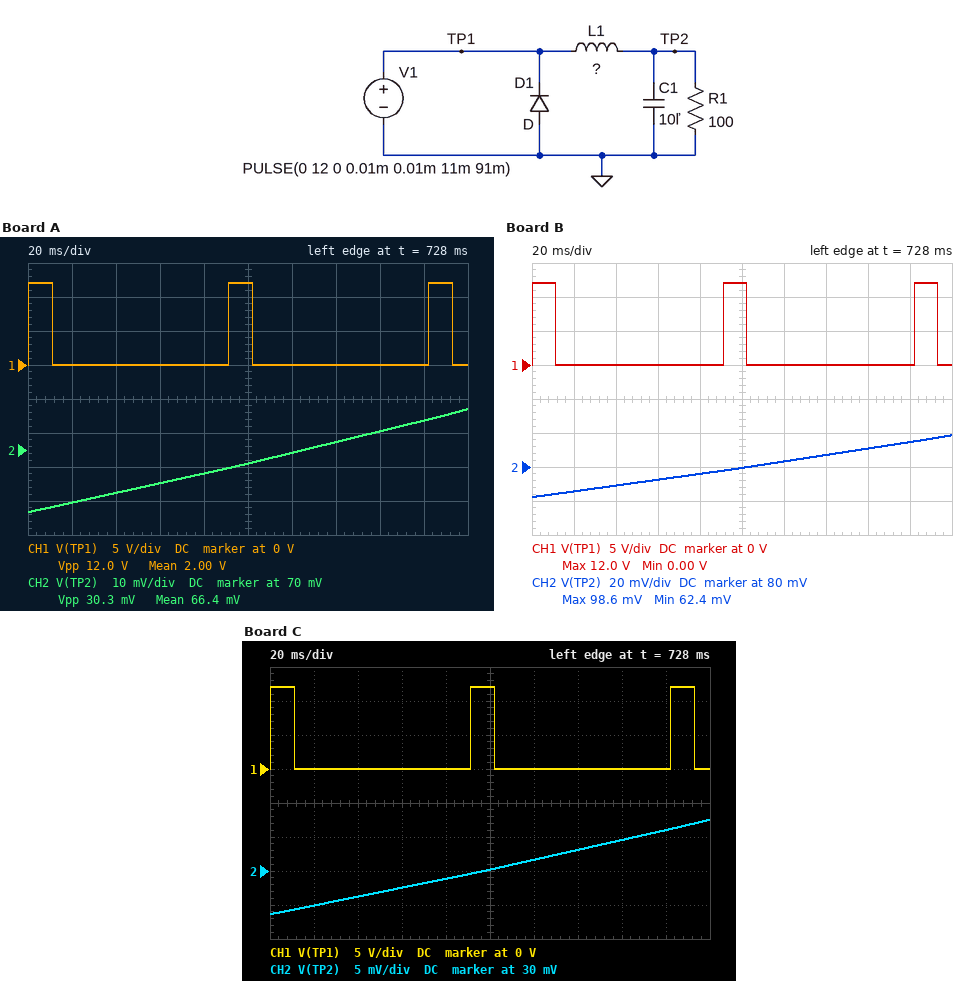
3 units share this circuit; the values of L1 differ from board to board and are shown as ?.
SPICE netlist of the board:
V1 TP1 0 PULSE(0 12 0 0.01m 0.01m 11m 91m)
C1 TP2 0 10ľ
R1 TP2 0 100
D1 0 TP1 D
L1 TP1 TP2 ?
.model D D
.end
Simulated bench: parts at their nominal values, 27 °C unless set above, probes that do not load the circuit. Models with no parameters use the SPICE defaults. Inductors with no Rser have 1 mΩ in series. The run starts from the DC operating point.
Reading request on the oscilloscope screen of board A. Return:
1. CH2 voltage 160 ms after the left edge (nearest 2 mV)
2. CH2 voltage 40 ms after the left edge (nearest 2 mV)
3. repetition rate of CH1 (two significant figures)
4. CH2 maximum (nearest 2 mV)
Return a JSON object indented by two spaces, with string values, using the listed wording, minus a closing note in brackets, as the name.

{
  "CH2 voltage 160 ms after the left edge": "76 mV",
  "CH2 voltage 40 ms after the left edge": "58 mV",
  "repetition rate of CH1": "11 Hz",
  "CH2 maximum": "82 mV"
}
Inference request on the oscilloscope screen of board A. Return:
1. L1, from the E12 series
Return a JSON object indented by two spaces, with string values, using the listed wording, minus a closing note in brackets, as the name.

{
  "L1, from the E12 series": "820 mH"
}
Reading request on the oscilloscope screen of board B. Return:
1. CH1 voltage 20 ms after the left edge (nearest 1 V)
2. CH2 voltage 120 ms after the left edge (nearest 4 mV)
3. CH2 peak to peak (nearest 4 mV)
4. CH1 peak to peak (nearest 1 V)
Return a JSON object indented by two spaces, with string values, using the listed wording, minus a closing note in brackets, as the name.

{
  "CH1 voltage 20 ms after the left edge": "0 V",
  "CH2 voltage 120 ms after the left edge": "84 mV",
  "CH2 peak to peak": "36 mV",
  "CH1 peak to peak": "12 V"
}
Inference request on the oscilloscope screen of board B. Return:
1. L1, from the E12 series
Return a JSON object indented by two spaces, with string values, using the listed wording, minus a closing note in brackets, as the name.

{
  "L1, from the E12 series": "680 mH"
}
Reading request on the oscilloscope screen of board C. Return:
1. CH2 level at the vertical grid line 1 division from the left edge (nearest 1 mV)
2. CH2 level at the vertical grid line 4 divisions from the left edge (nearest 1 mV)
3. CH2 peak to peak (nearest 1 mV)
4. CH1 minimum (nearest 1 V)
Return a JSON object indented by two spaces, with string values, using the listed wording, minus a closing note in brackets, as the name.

{
  "CH2 level at the vertical grid line 1 division from the left edge": "25 mV",
  "CH2 level at the vertical grid line 4 divisions from the left edge": "29 mV",
  "CH2 peak to peak": "14 mV",
  "CH1 minimum": "0 V"
}
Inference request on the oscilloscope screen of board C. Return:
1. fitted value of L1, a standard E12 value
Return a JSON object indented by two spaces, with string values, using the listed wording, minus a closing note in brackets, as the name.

{
  "fitted value of L1, a standard E12 value": "1.8 H"
}
